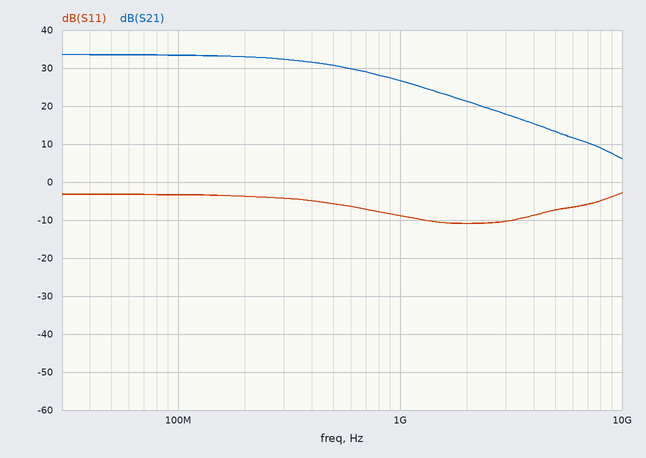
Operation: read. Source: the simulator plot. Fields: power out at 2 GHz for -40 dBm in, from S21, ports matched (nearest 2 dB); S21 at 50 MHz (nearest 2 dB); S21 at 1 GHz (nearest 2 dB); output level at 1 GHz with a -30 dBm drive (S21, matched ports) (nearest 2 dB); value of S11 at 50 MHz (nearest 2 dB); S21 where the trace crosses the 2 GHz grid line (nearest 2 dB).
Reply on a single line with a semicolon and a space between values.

-18 dBm; 34 dB; 26 dB; -4 dBm; -4 dB; 22 dB
